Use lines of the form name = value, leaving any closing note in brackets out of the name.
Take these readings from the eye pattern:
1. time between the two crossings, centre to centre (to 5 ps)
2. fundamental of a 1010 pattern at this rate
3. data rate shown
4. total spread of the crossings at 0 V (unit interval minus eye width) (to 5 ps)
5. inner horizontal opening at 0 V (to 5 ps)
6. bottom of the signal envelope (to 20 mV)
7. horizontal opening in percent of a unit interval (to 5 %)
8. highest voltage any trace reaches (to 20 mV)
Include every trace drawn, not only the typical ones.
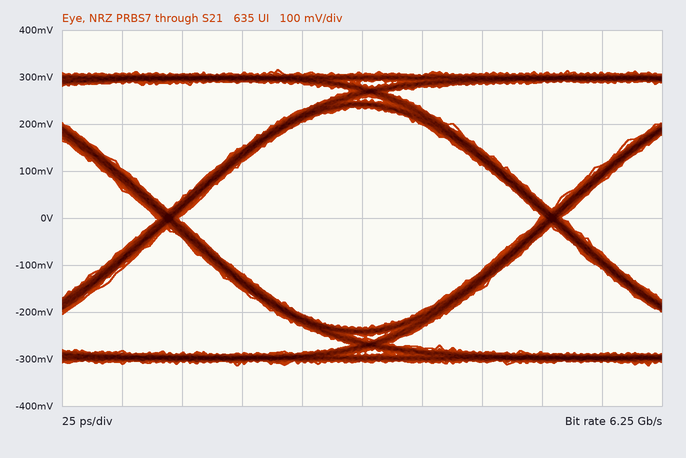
time between the two crossings, centre to centre = 160 ps
fundamental of a 1010 pattern at this rate = 3.125 GHz
data rate shown = 6.25 Gb/s
total spread of the crossings at 0 V (unit interval minus eye width) = 10 ps
inner horizontal opening at 0 V = 150 ps
bottom of the signal envelope = -320 mV
horizontal opening in percent of a unit interval = 95 %
highest voltage any trace reaches = 320 mV
